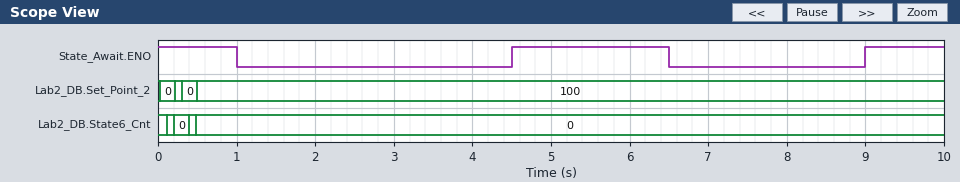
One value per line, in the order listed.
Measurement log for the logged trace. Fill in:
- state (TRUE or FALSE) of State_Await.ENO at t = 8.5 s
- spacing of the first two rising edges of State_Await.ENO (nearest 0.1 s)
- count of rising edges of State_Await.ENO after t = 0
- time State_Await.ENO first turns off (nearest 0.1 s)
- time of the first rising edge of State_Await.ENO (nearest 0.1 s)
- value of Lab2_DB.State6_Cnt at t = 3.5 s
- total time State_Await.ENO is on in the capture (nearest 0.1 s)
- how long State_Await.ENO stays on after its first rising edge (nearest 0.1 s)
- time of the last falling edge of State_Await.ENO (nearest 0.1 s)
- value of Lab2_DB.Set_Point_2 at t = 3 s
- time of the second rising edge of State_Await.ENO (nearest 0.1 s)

FALSE
4.5 s
2
1.0 s
4.5 s
0
4.0 s
2.0 s
6.5 s
100
9.0 s
